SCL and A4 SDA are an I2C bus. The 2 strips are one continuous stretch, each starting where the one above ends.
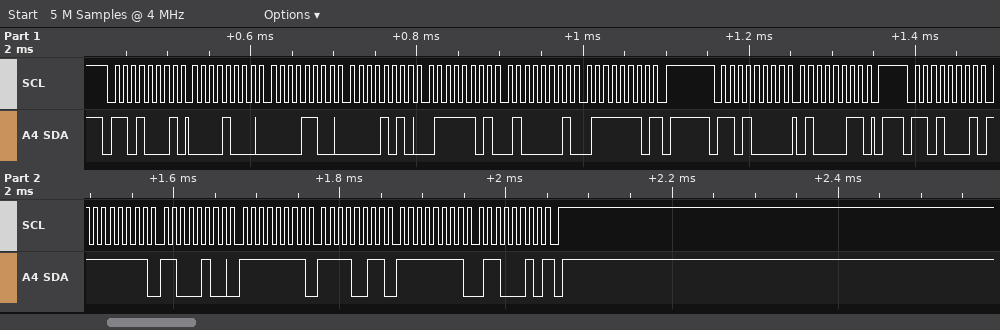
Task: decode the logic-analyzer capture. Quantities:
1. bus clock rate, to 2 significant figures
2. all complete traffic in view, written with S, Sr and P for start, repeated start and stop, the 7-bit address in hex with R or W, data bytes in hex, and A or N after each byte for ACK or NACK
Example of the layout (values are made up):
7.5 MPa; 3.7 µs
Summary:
100 kHz; S 68R A 08 A 0C A 0A A 7D A 41 A 7E N P S 68W A 43 A P S 68R A FF A C4 A FF A F3 A FF A 62 N P
